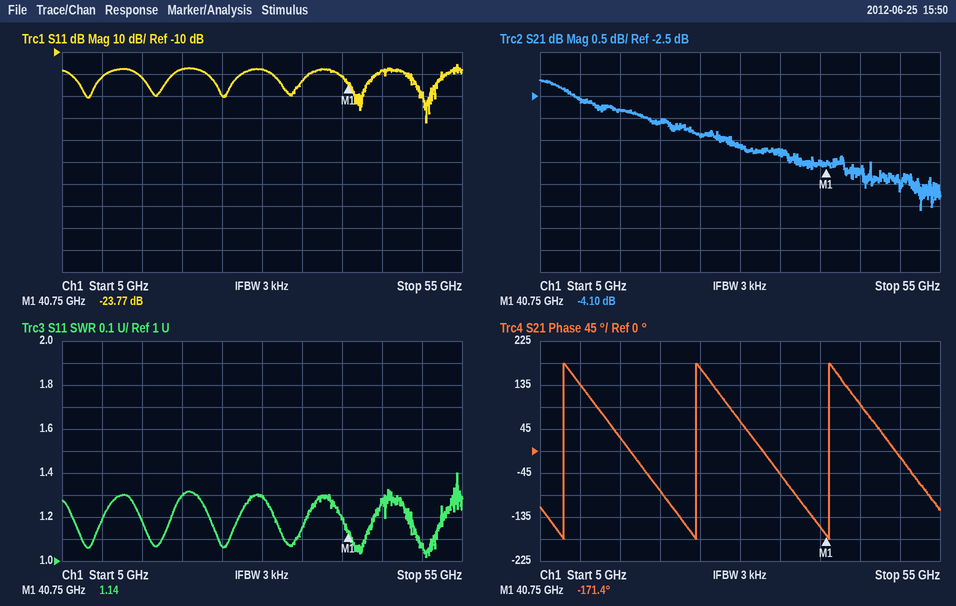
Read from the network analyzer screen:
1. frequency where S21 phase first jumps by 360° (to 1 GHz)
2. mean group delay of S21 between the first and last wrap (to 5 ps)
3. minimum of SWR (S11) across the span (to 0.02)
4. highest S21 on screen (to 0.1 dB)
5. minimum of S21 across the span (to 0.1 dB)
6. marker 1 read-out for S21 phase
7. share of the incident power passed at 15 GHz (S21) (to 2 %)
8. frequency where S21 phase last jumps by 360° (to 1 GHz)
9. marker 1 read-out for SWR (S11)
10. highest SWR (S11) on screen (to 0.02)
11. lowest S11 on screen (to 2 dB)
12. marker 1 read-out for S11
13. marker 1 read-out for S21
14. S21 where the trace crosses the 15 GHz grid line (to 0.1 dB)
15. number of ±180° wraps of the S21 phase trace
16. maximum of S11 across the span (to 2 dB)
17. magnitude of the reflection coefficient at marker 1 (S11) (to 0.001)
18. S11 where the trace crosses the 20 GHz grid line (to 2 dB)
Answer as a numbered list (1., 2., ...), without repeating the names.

1. 8 GHz
2. 60 ps
3. 1.02
4. -2.1 dB
5. -5.1 dB
6. -171.4°
7. 52 %
8. 41 GHz
9. 1.14
10. 1.40
11. -42 dB
12. -23.77 dB
13. -4.10 dB
14. -2.8 dB
15. 3
16. -16 dB
17. 0.065
18. -18 dB
